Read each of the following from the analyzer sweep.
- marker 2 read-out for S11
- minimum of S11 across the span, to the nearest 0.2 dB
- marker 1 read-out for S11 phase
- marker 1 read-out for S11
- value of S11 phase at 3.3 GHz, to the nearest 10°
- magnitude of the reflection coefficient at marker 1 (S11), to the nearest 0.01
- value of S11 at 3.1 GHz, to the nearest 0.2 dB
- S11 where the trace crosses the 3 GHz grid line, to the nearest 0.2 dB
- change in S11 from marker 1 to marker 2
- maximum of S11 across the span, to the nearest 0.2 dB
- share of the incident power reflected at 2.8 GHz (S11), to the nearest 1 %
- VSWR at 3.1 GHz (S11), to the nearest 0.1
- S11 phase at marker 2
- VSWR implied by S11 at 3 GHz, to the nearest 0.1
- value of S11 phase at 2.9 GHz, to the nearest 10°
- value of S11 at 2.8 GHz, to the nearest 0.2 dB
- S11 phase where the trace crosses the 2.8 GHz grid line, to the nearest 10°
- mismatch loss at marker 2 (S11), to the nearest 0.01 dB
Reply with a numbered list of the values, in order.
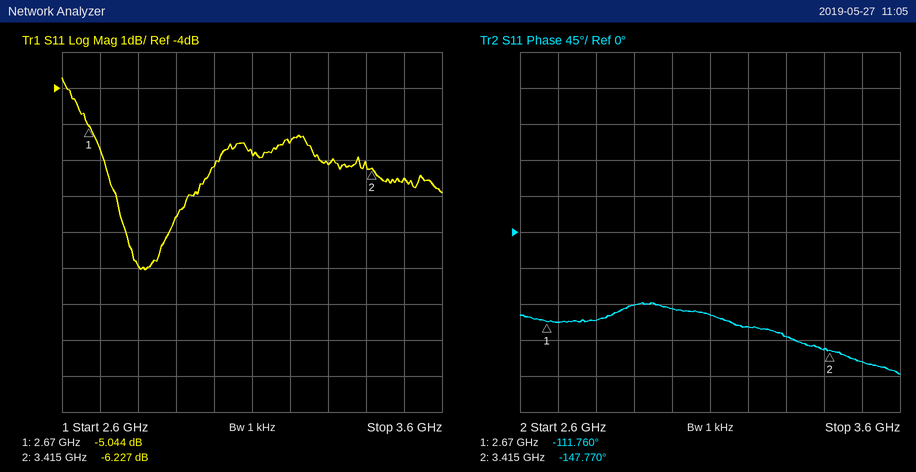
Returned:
1. -6.227 dB
2. -9.0 dB
3. -111.760°
4. -5.044 dB
5. -130°
6. 0.56
7. -5.8 dB
8. -6.2 dB
9. -1.183 dB
10. -3.8 dB
11. 13 %
12. 3.1
13. -147.770°
14. 2.9
15. -90°
16. -9.0 dB
17. -110°
18. 1.18 dB
